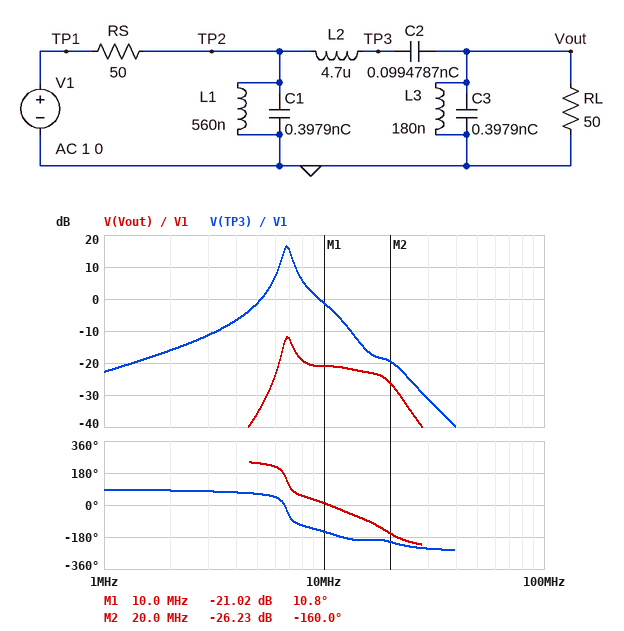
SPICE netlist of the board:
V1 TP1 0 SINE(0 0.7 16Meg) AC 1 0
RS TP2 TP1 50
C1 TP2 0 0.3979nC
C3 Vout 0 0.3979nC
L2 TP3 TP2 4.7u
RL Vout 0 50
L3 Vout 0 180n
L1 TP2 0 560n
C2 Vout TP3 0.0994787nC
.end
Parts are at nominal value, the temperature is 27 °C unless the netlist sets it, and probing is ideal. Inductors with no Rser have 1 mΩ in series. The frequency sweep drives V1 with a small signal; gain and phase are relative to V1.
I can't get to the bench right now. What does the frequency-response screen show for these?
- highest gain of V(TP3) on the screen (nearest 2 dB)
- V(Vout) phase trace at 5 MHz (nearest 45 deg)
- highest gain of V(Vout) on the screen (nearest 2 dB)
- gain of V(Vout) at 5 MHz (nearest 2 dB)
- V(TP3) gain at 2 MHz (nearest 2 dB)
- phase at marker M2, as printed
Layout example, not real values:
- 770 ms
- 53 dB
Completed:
- 16 dB
- 225 deg
- -12 dB
- -36 dB
- -16 dB
- -160.0 deg
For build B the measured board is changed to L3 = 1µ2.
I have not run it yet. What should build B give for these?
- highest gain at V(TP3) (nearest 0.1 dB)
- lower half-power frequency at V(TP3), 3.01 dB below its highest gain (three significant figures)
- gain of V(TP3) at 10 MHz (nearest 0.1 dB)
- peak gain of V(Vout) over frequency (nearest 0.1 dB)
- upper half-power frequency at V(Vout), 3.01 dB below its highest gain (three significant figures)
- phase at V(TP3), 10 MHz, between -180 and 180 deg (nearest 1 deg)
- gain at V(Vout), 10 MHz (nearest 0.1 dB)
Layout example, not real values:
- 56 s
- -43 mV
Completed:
- 6.6 dB
- 5.77 MHz
- 1.8 dB
- -6.8 dB
- 9.34 MHz
- -124 deg
- -10.9 dB
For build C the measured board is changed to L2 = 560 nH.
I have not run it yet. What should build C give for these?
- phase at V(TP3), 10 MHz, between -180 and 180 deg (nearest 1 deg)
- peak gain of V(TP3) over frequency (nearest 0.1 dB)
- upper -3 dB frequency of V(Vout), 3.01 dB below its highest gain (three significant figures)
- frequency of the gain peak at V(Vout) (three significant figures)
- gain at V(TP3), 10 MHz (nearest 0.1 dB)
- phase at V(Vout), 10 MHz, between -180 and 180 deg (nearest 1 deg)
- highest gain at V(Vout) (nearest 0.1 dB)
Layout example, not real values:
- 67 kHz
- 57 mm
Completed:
- -16 deg
- 3.7 dB
- 29.2 MHz
- 27.3 MHz
- 1.9 dB
- 145 deg
- -6.7 dB
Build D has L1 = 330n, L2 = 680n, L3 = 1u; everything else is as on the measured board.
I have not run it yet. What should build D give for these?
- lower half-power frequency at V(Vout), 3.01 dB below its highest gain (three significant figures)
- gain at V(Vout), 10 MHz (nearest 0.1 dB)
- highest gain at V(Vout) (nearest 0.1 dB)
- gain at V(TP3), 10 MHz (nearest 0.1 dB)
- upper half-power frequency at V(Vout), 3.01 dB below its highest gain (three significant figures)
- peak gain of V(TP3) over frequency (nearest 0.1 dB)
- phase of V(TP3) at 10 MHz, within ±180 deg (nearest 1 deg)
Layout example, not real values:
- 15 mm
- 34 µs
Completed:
- 21.8 MHz
- -12.7 dB
- -6.3 dB
- -0.6 dB
- 25.7 MHz
- 7.3 dB
- 33 deg
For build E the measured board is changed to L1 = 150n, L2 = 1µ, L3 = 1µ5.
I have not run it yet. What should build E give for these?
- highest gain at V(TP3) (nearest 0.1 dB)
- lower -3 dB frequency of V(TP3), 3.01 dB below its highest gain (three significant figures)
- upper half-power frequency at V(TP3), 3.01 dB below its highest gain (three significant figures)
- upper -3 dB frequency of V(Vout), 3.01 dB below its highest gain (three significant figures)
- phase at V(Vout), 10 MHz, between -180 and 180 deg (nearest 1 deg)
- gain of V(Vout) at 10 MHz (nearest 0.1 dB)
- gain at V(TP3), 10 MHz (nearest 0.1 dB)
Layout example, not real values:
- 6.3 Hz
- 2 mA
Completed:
- 7.5 dB
- 14.3 MHz
- 18.3 MHz
- 18.2 MHz
- 112 deg
- -21.5 dB
- -8.2 dB
